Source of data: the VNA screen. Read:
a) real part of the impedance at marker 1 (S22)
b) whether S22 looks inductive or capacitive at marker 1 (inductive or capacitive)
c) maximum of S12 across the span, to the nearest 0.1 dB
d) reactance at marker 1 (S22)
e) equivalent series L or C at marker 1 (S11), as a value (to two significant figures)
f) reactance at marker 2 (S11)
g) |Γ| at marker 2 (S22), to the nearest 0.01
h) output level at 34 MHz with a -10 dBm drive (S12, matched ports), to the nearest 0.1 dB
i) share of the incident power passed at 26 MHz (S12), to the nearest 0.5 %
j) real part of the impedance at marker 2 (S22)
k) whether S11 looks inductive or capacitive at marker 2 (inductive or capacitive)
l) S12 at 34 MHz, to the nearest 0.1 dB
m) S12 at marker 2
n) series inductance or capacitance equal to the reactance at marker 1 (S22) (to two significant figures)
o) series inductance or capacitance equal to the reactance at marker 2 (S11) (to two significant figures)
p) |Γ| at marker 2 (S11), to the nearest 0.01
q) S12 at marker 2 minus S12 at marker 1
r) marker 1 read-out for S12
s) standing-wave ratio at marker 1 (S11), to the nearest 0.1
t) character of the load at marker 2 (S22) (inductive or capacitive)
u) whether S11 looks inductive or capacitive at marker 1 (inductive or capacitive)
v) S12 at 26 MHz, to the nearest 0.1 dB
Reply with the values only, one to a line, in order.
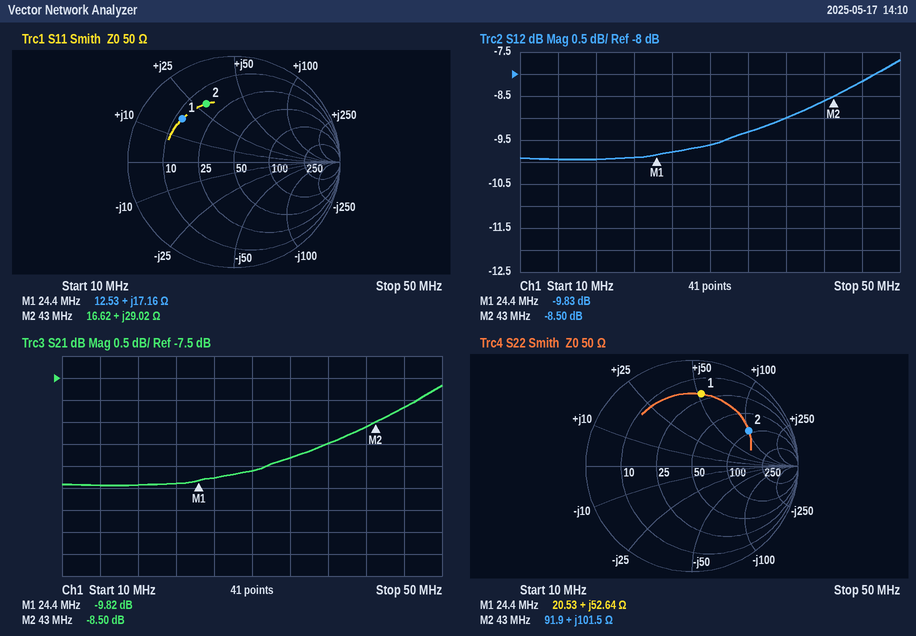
20.53 Ω
inductive
-7.7 dB
+52.64 Ω
110 nH
+29.02 Ω
0.63
-19.3 dBm
10.5 %
91.9 Ω
inductive
-9.3 dB
-8.50 dB
340 nH
110 nH
0.61
1.33 dB
-9.83 dB
4.5
inductive
inductive
-9.8 dB
